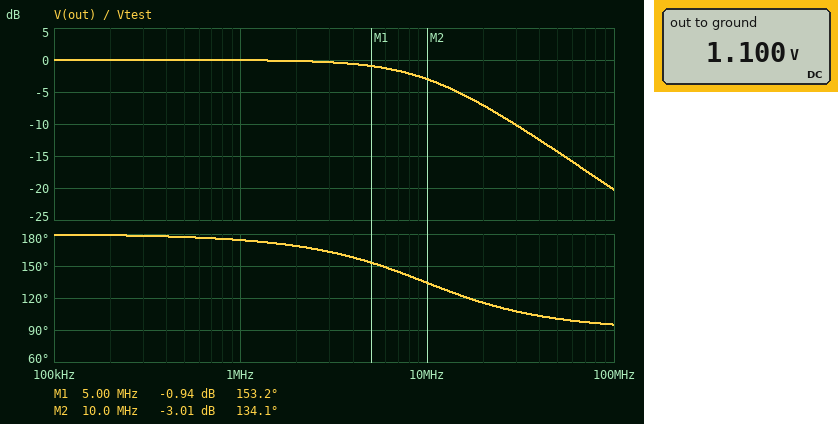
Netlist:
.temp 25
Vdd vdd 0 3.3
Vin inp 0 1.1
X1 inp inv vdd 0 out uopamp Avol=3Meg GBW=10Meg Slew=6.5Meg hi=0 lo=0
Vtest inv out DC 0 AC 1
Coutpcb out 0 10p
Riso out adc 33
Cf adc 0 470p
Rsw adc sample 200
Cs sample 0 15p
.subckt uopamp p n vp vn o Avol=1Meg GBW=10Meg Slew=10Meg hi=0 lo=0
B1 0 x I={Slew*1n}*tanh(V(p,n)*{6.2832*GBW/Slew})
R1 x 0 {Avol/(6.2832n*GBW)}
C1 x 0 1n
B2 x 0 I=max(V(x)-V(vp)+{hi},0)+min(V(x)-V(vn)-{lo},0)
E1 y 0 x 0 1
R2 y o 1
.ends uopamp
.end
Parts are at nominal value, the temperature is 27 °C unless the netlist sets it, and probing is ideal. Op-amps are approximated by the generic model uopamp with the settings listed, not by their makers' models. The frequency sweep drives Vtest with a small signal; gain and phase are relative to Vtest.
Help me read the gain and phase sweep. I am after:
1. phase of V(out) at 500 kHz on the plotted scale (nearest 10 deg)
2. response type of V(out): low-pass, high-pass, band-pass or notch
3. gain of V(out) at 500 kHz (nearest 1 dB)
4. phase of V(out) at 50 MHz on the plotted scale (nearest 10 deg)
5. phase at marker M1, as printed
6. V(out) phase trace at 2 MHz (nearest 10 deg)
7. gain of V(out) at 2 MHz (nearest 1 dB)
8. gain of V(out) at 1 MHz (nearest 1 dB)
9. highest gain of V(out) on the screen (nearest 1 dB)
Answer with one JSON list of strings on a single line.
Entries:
["180 deg", "low-pass", "0 dB", "100 deg", "153.2 deg", "170 deg", "0 dB", "0 dB", "0 dB"]
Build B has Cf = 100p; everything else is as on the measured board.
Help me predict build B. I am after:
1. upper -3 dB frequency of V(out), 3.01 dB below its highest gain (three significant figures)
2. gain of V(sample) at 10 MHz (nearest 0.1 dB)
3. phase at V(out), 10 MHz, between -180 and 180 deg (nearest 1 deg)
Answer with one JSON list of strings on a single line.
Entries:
["10.1 MHz", "-3.4 dB", "135 deg"]
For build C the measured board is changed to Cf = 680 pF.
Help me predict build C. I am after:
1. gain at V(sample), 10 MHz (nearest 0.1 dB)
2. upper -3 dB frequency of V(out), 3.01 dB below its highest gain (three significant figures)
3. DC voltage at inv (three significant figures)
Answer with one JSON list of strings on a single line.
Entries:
["-8.1 dB", "9.94 MHz", "1.10 V"]
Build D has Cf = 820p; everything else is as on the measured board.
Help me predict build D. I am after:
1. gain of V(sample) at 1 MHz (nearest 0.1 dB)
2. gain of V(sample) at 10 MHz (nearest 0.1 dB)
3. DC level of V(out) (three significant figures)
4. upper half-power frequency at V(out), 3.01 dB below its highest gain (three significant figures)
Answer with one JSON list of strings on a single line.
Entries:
["-0.2 dB", "-9.2 dB", "1.10 V", "9.91 MHz"]
